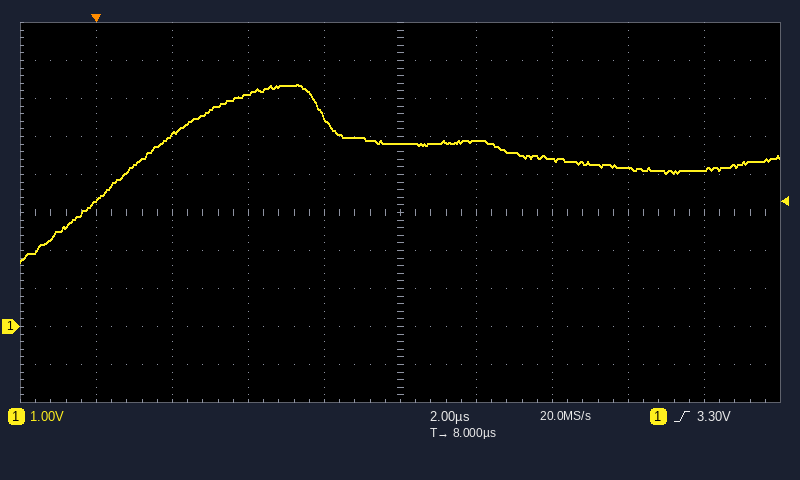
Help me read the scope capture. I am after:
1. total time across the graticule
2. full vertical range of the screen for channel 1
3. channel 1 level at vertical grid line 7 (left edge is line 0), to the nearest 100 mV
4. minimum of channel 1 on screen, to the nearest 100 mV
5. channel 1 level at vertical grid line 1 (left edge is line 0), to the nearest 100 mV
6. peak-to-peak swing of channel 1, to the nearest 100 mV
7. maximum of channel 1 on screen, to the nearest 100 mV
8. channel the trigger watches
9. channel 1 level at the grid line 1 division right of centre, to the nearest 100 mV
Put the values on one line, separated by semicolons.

20 µs; 10 V; 4.4 V; 1.7 V; 3.3 V; 4.7 V; 6.4 V; channel 1; 4.9 V
